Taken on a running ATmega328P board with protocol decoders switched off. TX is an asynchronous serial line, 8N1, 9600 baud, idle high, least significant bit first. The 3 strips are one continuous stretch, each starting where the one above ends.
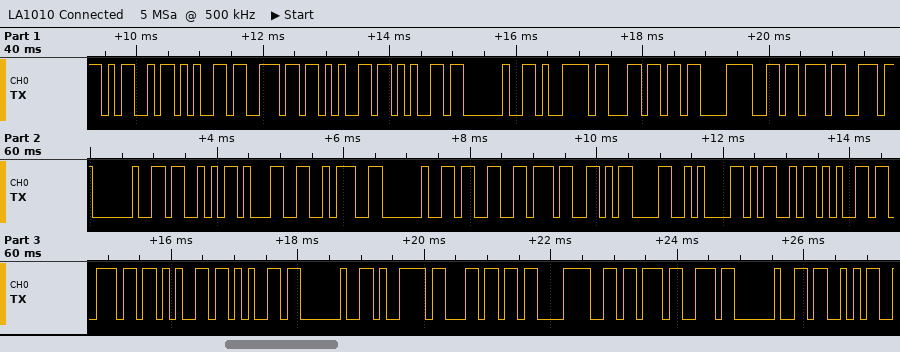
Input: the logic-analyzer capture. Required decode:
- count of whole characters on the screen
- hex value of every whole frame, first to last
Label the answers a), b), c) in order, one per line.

a) 33
b) 4D 65 6E 65 65 20 79 6C C3 B6 73 20 53 31 3A 20 33 37 0D 0A 4D 65 6E 65 65 20 79 6C C3 B6 73 20 53
